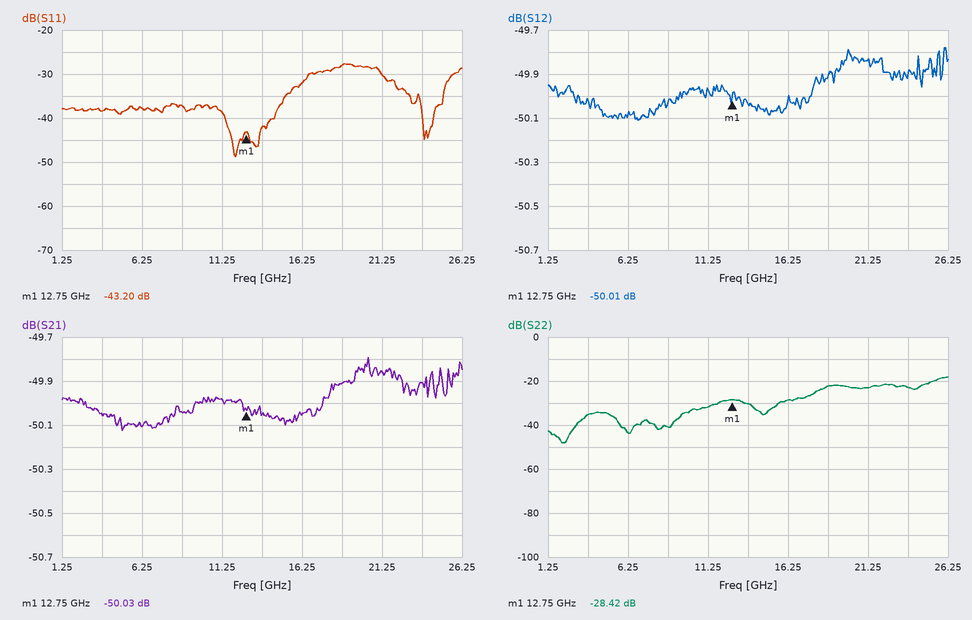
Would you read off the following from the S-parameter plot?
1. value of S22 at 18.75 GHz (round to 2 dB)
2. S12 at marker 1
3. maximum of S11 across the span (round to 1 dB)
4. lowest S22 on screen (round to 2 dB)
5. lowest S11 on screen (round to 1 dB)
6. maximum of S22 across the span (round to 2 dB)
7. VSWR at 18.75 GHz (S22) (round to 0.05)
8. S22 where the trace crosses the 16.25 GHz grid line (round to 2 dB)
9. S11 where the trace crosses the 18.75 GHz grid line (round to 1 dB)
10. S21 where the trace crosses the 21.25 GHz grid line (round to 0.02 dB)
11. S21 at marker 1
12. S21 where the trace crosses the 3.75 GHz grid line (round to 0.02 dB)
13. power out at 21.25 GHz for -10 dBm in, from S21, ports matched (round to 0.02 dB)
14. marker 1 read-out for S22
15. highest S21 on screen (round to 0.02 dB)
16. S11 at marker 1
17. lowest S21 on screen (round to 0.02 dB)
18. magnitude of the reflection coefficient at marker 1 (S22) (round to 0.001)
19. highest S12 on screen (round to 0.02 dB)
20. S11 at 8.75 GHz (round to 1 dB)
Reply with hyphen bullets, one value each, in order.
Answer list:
- -22 dB
- -50.01 dB
- -28 dB
- -48 dB
- -49 dB
- -18 dB
- 1.15
- -28 dB
- -28 dB
- -49.86 dB
- -50.03 dB
- -50.06 dB
- -59.86 dBm
- -28.42 dB
- -49.80 dB
- -43.20 dB
- -50.12 dB
- 0.038
- -49.78 dB
- -37 dB
